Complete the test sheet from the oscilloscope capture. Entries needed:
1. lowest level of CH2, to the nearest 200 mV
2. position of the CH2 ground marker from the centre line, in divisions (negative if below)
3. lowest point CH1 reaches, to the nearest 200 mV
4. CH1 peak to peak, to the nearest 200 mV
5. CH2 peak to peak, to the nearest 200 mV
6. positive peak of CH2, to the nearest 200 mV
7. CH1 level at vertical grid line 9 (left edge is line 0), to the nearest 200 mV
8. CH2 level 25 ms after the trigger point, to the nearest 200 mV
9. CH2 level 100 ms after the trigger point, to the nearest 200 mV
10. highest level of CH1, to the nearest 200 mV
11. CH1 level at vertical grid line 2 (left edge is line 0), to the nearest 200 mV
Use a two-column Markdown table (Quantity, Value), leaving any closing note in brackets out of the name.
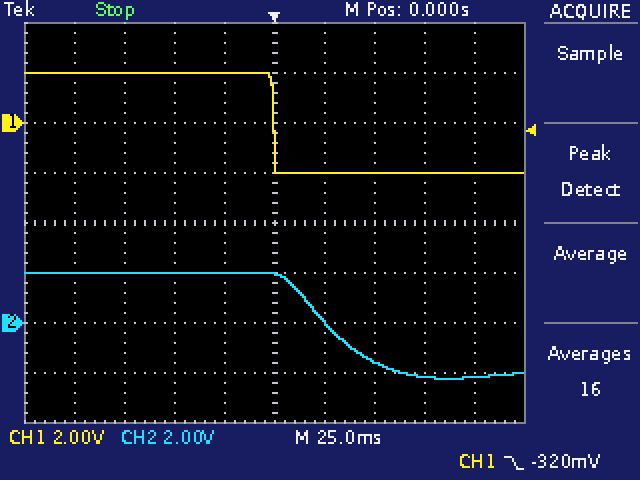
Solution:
| Quantity | Value |
|---|---|
| lowest level of CH2, to the nearest 200 mV | -2.2 V |
| position of the CH2 ground marker from the centre line, in divisions | -2.0 div |
| lowest point CH1 reaches, to the nearest 200 mV | -2.0 V |
| CH1 peak to peak, to the nearest 200 mV | 4.0 V |
| CH2 peak to peak, to the nearest 200 mV | 4.2 V |
| positive peak of CH2, to the nearest 200 mV | 2.0 V |
| CH1 level at vertical grid line 9 (left edge is line 0), to the nearest 200 mV | -2.0 V |
| CH2 level 25 ms after the trigger point, to the nearest 200 mV | 0.0 V |
| CH2 level 100 ms after the trigger point, to the nearest 200 mV | -2.2 V |
| highest level of CH1, to the nearest 200 mV | 2.0 V |
| CH1 level at vertical grid line 2 (left edge is line 0), to the nearest 200 mV | 2.0 V |
